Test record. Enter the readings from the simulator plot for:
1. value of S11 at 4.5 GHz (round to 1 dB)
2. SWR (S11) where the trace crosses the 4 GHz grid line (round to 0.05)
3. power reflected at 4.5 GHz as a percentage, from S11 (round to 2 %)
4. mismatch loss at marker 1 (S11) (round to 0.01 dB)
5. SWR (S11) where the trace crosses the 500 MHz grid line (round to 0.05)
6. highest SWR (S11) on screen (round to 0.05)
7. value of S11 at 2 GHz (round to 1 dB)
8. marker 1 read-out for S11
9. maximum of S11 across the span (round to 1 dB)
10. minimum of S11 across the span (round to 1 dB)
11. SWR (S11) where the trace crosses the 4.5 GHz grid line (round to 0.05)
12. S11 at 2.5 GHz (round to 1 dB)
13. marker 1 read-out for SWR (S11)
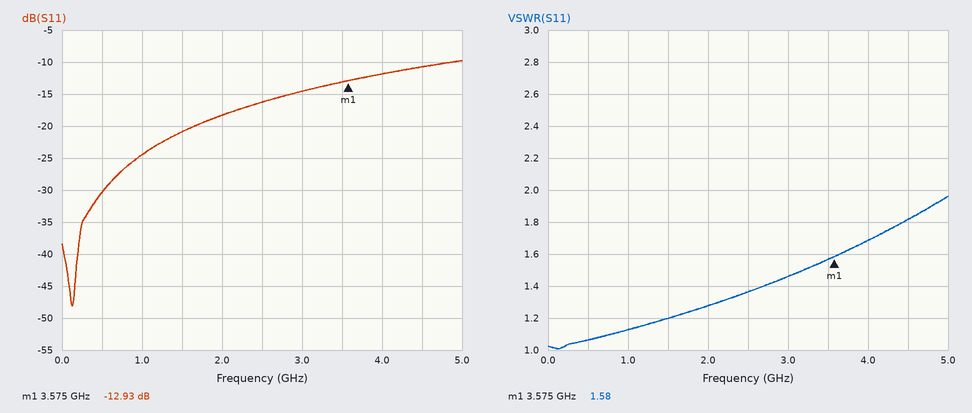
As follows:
-11 dB
1.70
8 %
0.23 dB
1.05
1.95
-18 dB
-12.93 dB
-10 dB
-48 dB
1.80
-16 dB
1.58
